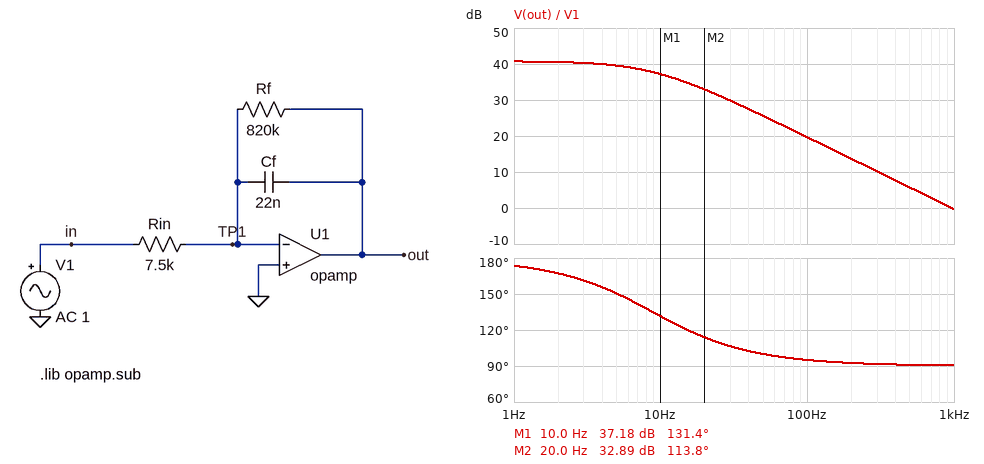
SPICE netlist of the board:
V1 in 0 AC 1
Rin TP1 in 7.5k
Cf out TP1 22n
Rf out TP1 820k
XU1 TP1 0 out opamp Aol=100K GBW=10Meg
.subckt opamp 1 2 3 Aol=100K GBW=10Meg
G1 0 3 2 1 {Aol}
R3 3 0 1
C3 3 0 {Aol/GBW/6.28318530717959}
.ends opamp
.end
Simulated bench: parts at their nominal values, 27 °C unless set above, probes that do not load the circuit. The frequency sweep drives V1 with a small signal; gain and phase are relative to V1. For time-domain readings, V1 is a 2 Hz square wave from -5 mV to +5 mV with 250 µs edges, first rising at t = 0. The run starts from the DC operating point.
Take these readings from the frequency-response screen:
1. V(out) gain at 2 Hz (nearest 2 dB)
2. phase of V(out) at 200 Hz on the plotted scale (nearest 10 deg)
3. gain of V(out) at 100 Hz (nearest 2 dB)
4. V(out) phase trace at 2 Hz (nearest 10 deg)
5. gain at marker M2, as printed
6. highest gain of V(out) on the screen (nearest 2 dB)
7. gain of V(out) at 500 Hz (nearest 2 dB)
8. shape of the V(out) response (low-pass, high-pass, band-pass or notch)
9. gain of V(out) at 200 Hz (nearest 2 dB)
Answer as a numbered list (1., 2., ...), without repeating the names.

1. 40 dB
2. 90 deg
3. 20 dB
4. 170 deg
5. 32.89 dB
6. 40 dB
7. 6 dB
8. low-pass
9. 14 dB
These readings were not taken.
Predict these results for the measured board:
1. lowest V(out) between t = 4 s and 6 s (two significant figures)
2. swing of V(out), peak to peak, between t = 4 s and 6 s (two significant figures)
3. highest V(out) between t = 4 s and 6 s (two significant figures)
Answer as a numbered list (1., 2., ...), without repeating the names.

1. -550 mV
2. 1.1 V
3. 550 mV
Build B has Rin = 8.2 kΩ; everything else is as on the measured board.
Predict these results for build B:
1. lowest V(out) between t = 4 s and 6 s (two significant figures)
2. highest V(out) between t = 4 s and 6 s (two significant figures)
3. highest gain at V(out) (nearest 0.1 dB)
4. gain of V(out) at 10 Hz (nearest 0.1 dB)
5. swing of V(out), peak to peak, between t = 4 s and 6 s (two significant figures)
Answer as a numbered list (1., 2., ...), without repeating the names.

1. -500 mV
2. 500 mV
3. 40.0 dB
4. 36.4 dB
5. 1.0 V
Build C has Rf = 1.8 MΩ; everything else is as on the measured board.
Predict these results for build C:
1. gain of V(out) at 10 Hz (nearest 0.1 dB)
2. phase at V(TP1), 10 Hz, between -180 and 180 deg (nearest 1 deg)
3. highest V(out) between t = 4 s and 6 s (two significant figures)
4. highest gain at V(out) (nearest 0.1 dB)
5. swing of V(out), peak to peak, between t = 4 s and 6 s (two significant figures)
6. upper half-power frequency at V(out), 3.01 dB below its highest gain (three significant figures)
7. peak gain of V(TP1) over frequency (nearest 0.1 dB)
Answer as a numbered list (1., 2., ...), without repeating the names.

1. 39.0 dB
2. -62 deg
3. 1.2 V
4. 47.6 dB
5. 2.4 V
6. 4.03 Hz
7. -52.4 dB
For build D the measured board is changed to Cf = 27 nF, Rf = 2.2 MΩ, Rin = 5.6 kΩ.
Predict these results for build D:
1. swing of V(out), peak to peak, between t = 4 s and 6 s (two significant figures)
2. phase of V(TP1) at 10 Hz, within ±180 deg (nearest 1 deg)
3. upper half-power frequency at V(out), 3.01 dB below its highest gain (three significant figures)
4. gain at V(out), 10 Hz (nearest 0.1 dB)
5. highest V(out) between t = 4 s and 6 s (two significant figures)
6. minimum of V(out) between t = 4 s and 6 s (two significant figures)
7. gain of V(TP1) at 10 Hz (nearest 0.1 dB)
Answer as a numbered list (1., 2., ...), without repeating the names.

1. 3.8 V
2. -69 deg
3. 2.69 Hz
4. 40.1 dB
5. 1.9 V
6. -1.9 V
7. -59.8 dB
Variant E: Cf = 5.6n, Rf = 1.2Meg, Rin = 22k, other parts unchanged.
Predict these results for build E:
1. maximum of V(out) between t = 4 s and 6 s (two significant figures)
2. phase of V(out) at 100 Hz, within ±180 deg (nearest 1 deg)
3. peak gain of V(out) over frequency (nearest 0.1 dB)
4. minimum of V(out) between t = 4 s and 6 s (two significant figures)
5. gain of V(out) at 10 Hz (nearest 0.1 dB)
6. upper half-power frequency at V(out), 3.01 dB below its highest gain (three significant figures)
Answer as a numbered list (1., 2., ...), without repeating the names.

1. 270 mV
2. 103 deg
3. 34.7 dB
4. -270 mV
5. 34.0 dB
6. 23.7 Hz
